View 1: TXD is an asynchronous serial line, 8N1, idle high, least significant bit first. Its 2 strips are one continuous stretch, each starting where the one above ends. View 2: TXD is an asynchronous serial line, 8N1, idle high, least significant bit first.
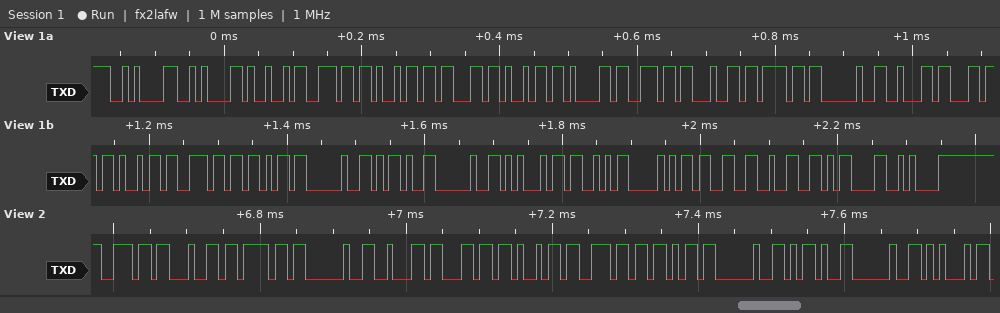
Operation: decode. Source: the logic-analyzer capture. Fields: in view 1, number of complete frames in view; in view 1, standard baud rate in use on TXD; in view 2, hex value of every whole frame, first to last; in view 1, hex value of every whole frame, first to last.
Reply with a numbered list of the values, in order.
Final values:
1. 27
2. 115200 baud
3. 6E 64 6F 20 62 6C 69 6E 6B 20 2D 20 45
4. 0A 0A 49 6E 69 63 69 61 6E 64 6F 20 62 6C 69 6E 6B 20 2D 20 45 53 50 33 32 0D 0A
